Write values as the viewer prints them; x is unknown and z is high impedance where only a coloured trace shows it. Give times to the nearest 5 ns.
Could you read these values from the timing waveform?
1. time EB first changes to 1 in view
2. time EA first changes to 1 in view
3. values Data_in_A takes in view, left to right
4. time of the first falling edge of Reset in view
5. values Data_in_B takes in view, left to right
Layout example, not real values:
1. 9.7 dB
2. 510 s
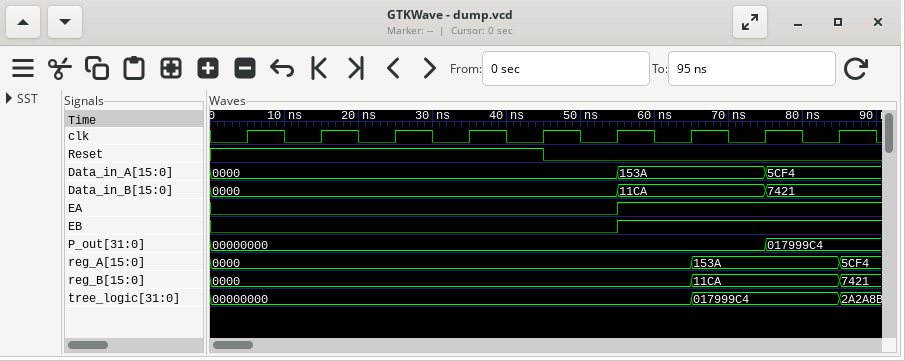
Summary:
1. 55 ns
2. 55 ns
3. 0000, 153A, 5CF4
4. 45 ns
5. 0000, 11CA, 7421
